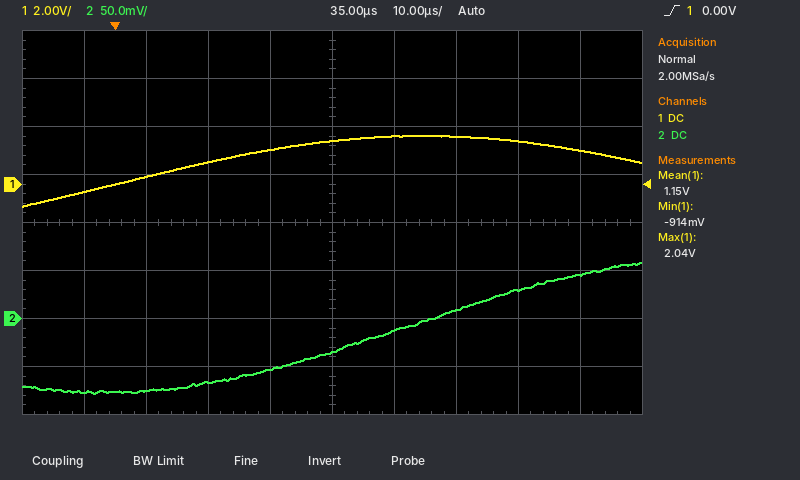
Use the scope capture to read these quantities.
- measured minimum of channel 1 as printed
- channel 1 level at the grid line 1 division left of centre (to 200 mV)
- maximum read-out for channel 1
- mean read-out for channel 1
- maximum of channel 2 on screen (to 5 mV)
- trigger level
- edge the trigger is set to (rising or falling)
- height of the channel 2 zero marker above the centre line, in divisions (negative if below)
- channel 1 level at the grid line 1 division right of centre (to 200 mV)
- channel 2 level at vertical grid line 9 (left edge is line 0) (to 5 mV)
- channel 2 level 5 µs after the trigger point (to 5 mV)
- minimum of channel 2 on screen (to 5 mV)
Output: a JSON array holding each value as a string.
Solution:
["-914 mV", "1.4 V", "2.04 V", "1.15 V", "60 mV", "0.00 V", "rising", "-2.0 div", "2.0 V", "45 mV", "-75 mV", "-80 mV"]
